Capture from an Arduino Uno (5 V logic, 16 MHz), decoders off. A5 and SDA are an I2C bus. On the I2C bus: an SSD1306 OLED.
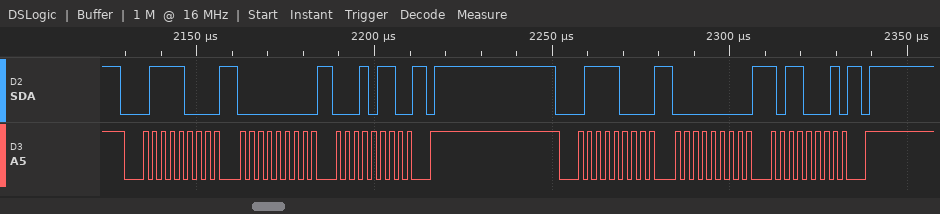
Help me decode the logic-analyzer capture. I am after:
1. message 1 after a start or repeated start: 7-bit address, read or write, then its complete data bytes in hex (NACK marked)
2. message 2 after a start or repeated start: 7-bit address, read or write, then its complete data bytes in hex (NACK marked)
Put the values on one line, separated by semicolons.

0x3C write: 00 16; 0x3C write: 00 B1
